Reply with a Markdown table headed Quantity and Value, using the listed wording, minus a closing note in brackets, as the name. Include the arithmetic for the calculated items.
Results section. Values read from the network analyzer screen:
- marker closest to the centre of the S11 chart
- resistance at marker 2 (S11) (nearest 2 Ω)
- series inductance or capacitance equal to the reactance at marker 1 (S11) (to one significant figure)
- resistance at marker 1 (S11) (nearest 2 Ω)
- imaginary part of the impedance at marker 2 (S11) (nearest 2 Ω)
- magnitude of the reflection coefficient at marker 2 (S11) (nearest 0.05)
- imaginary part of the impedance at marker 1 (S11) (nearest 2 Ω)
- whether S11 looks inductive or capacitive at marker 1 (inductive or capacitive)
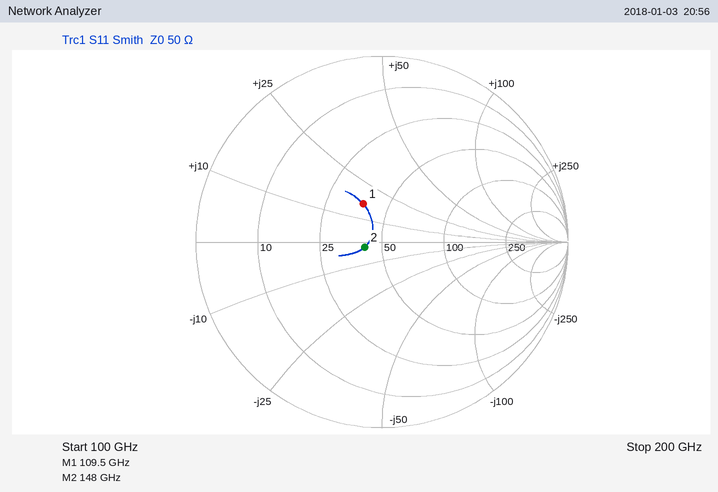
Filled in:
| Quantity | Value |
|---|---|
| marker closest to the centre of the S11 chart | marker 2 |
| resistance at marker 2 (S11) | 42 Ω |
| series inductance or capacitance equal to the reactance at marker 1 (S11) | L = 16 Ω/(2π × 109.5 GHz) ≈ 23.3 pH, so 20 pH to one significant figure |
| resistance at marker 1 (S11) | 38 Ω |
| imaginary part of the impedance at marker 2 (S11) | -2 Ω |
| magnitude of the reflection coefficient at marker 2 (S11) | 0.10 |
| imaginary part of the impedance at marker 1 (S11) | +16 Ω |
| whether S11 looks inductive or capacitive at marker 1 | inductive |
